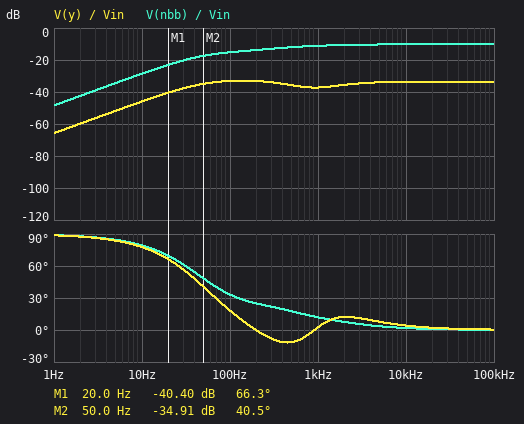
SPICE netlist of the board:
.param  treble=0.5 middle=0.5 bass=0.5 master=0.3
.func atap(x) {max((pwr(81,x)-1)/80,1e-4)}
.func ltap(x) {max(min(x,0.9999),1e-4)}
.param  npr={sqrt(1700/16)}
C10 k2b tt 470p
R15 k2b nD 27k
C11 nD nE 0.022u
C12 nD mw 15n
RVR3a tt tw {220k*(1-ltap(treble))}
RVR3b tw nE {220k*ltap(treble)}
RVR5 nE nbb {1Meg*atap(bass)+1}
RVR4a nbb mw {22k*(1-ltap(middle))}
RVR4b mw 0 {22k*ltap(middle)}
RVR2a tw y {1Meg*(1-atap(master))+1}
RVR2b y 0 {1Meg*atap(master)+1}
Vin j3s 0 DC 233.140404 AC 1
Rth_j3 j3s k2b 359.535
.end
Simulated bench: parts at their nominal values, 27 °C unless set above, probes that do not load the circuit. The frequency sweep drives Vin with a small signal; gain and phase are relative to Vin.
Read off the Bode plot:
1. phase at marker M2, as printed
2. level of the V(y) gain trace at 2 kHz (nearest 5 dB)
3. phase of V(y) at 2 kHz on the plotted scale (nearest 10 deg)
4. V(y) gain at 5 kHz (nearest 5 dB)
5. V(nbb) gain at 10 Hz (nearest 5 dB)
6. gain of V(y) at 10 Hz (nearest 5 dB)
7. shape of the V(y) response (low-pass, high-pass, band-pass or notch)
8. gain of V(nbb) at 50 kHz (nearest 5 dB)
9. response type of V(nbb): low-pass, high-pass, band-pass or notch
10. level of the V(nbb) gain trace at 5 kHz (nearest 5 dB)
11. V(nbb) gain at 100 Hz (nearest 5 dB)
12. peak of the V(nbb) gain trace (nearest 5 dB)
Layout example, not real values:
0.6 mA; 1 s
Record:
40.5 deg; -35 dB; 10 deg; -35 dB; -30 dB; -45 dB; high-pass; -10 dB; high-pass; -10 dB; -15 dB; -10 dB
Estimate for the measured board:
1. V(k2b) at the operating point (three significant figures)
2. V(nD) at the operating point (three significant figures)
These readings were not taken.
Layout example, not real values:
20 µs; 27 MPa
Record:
233 V; 233 V
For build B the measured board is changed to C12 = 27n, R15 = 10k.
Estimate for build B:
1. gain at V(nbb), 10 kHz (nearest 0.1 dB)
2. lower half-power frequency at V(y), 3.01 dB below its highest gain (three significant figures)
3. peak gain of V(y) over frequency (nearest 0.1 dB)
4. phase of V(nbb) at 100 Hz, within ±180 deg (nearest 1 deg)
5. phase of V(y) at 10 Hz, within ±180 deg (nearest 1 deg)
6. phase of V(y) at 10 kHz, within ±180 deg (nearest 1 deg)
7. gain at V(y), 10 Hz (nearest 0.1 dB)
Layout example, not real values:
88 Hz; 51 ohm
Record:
-5.6 dB; 45.2 Hz; -31.4 dB; 43 deg; 79 deg; 3 deg; -45.5 dB
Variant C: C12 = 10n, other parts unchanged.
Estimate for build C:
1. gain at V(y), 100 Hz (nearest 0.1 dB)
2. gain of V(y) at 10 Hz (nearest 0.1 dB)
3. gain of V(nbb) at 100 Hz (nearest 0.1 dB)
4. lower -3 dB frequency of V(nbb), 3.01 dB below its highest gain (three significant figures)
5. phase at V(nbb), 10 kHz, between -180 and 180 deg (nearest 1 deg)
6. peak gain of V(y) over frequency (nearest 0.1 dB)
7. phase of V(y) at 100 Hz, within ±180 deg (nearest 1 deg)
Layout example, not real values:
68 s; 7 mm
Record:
-33.0 dB; -46.1 dB; -15.9 dB; 428 Hz; 2 deg; -32.6 dB; 21 deg
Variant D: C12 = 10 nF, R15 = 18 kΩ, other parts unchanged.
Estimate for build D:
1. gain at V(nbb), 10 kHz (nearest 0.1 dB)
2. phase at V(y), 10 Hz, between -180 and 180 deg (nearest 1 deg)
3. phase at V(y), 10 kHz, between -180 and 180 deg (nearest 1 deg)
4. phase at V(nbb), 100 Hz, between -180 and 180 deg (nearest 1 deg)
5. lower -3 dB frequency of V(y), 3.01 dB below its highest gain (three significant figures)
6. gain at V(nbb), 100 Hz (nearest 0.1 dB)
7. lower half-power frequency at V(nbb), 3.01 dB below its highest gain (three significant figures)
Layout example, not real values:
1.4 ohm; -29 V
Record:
-8.2 dB; 79 deg; 3 deg; 36 deg; 47.4 Hz; -15.4 dB; 576 Hz
